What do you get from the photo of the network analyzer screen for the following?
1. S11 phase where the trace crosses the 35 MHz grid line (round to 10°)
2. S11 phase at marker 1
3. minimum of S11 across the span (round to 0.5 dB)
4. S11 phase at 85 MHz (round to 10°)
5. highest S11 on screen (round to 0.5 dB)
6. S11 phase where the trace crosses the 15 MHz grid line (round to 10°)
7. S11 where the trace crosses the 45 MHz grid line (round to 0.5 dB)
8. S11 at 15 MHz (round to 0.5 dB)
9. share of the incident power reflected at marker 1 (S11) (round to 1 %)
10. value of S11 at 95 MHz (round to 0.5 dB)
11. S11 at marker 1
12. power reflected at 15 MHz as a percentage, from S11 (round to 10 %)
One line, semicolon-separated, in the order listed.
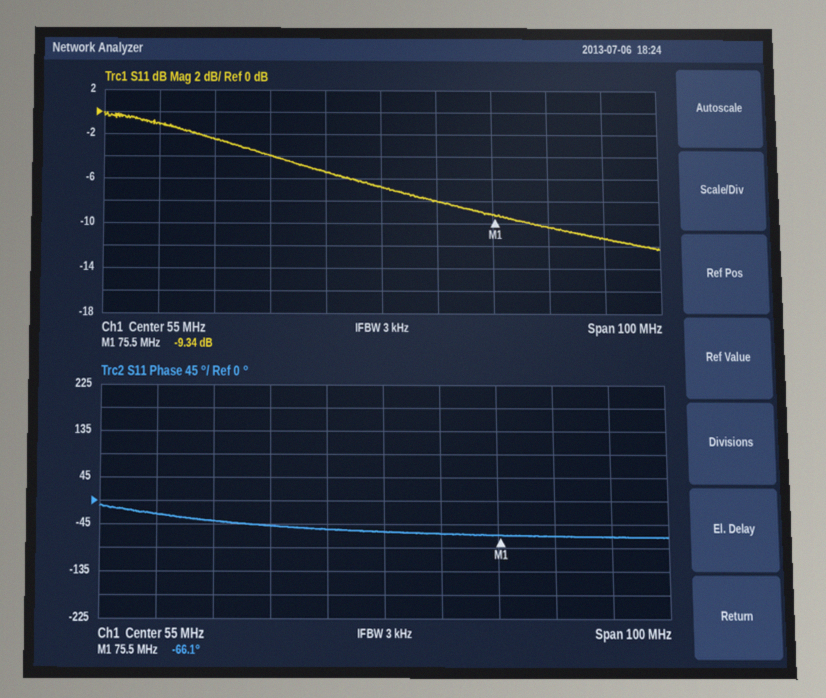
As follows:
-50°; -66.1°; -12.5 dB; -70°; 0.0 dB; -30°; -5.5 dB; -1.0 dB; 12 %; -11.5 dB; -9.34 dB; 80 %
